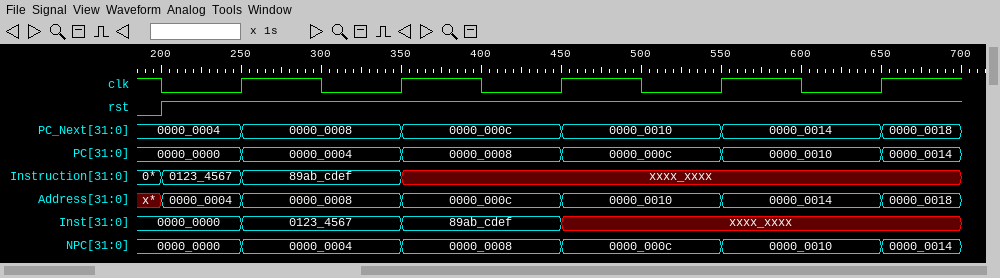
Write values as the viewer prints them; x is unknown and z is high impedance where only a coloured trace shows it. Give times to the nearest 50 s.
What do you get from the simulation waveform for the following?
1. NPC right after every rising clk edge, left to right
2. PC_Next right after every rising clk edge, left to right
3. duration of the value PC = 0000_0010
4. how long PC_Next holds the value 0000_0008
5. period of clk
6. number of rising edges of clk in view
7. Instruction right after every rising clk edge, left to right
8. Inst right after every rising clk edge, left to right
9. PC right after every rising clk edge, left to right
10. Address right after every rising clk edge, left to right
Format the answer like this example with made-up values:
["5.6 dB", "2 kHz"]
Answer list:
["0000_0004, 0000_0008, 0000_000c, 0000_0010, 0000_0014", "0000_0008, 0000_000c, 0000_0010, 0000_0014, 0000_0018", "100 s", "100 s", "100 s", "5", "89ab_cdef, xxxx_xxxx, xxxx_xxxx, xxxx_xxxx, xxxx_xxxx", "0123_4567, 89ab_cdef, xxxx_xxxx, xxxx_xxxx, xxxx_xxxx", "0000_0004, 0000_0008, 0000_000c, 0000_0010, 0000_0014", "0000_0008, 0000_000c, 0000_0010, 0000_0014, 0000_0018"]
